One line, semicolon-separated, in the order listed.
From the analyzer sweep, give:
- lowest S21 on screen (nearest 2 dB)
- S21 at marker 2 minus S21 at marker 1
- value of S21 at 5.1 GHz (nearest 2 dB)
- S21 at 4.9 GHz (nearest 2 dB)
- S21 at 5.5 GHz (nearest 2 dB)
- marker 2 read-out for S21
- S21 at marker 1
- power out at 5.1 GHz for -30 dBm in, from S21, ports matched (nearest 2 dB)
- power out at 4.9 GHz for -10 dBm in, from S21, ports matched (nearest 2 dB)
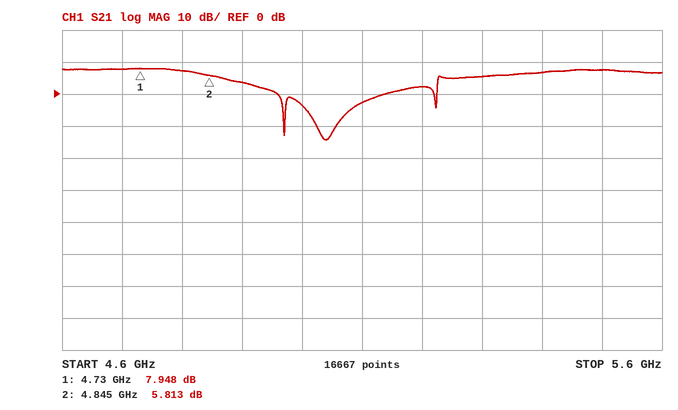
-14 dB; -2.135 dB; -2 dB; 4 dB; 8 dB; 5.813 dB; 7.948 dB; -32 dBm; -6 dBm
